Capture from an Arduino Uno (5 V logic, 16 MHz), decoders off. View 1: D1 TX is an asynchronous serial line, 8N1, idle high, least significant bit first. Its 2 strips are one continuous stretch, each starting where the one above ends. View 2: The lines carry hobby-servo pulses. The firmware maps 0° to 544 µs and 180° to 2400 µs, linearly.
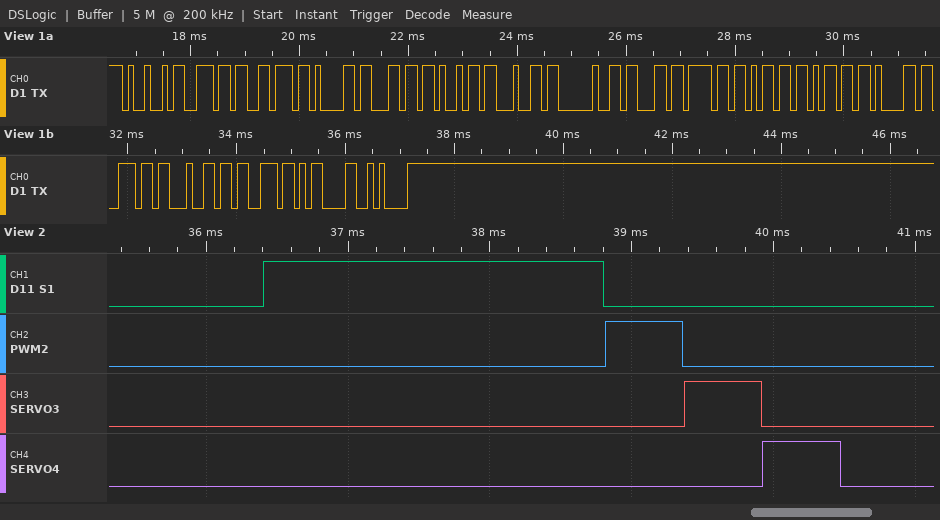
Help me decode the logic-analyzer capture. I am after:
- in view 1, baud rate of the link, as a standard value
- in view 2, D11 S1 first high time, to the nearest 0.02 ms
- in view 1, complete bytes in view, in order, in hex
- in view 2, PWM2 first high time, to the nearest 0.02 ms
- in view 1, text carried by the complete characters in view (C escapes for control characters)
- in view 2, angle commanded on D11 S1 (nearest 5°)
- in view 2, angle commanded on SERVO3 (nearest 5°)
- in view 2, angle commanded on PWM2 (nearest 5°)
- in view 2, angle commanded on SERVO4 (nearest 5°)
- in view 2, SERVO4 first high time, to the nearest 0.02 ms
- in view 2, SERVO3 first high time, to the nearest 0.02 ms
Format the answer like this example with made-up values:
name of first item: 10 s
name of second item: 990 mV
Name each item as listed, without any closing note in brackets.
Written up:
in view 1, baud rate of the link, as a standard value: 9600 baud
in view 2, D11 S1 first high time, to the nearest 0.02 ms: 2.40 ms
in view 1, complete bytes in view, in order, in hex: 49 6E 76 61 6C 69 64 20 63 6F 6D 6D 61 6E 64 73 0D 0A
in view 2, PWM2 first high time, to the nearest 0.02 ms: 0.54 ms
in view 1, text carried by the complete characters in view: "Invalid commands\r\n"
in view 2, angle commanded on D11 S1: 180°
in view 2, angle commanded on SERVO3: 0°
in view 2, angle commanded on PWM2: 0°
in view 2, angle commanded on SERVO4: 0°
in view 2, SERVO4 first high time, to the nearest 0.02 ms: 0.54 ms
in view 2, SERVO3 first high time, to the nearest 0.02 ms: 0.54 ms
